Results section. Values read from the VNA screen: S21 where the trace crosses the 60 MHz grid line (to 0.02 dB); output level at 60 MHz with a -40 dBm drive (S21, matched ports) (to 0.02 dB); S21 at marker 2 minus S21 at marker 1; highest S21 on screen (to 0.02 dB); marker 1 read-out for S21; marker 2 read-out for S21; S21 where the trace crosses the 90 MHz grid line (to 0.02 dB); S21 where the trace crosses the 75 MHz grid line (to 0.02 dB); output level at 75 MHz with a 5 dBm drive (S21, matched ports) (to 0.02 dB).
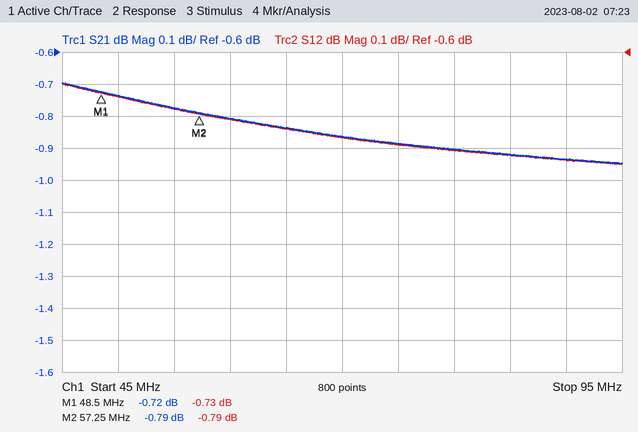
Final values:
-0.80 dB
-40.80 dBm
-0.07 dB
-0.70 dB
-0.72 dB
-0.79 dB
-0.94 dB
-0.88 dB
4.12 dBm
